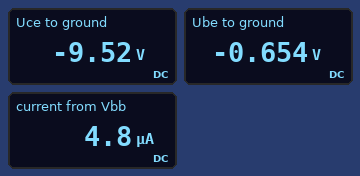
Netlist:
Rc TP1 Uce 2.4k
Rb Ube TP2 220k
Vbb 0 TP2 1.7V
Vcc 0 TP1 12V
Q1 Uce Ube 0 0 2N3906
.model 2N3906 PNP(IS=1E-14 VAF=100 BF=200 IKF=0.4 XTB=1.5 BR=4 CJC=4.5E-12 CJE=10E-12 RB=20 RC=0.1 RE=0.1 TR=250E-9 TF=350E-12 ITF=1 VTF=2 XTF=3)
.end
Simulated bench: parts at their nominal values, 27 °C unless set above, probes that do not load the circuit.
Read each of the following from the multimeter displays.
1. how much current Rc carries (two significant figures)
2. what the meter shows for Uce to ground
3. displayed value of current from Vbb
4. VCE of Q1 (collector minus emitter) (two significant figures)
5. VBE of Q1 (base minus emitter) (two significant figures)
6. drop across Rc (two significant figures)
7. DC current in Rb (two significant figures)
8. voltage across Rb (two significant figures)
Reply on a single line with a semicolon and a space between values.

1.0 mA; -9.52 V; 4.8 µA; -9.5 V; -650 mV; 2.5 V; 4.8 µA; 1.0 V
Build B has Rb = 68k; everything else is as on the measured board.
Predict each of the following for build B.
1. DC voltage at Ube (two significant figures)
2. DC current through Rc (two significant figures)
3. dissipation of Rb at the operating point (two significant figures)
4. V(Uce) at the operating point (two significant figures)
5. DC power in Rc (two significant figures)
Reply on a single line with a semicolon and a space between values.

-680 mV; 3.1 mA; 15 µW; -4.6 V; 23 mW
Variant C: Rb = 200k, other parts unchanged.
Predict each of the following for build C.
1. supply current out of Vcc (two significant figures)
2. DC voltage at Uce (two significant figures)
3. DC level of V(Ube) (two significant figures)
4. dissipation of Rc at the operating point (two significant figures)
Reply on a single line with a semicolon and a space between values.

1.1 mA; -9.3 V; -660 mV; 3.1 mW
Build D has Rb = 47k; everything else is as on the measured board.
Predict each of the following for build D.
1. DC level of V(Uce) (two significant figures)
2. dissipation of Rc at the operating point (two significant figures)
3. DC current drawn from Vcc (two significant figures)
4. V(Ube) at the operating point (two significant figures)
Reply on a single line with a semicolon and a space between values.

-1.7 V; 44 mW; 4.3 mA; -690 mV
